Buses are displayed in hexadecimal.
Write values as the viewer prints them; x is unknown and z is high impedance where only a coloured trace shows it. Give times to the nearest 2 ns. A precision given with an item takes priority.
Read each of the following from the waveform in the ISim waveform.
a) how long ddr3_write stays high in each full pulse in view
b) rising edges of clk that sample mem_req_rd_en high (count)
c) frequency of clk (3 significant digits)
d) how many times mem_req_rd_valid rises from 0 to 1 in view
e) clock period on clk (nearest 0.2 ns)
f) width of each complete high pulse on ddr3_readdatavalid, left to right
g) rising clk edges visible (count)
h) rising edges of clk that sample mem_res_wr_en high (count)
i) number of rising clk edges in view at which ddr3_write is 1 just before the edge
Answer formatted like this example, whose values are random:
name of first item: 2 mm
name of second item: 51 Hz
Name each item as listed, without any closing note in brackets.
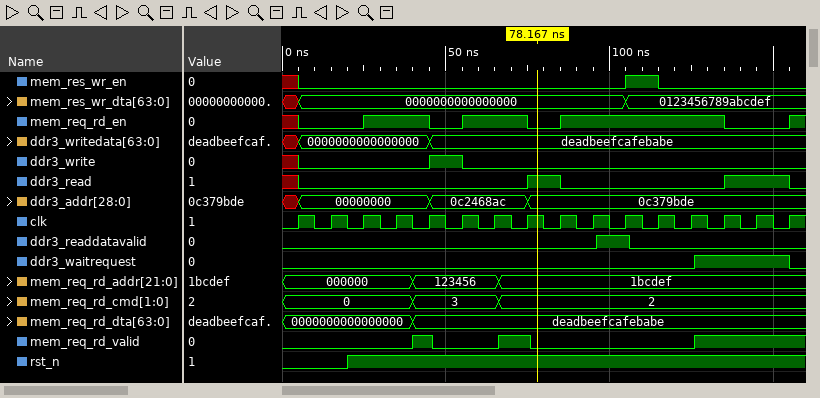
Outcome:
how long ddr3_write stays high in each full pulse in view: 10 ns
rising edges of clk that sample mem_req_rd_en high: 9
frequency of clk: 100 MHz
how many times mem_req_rd_valid rises from 0 to 1 in view: 3
clock period on clk: 10 ns
width of each complete high pulse on ddr3_readdatavalid, left to right: 10 ns
rising clk edges visible: 16
rising edges of clk that sample mem_res_wr_en high: 1
number of rising clk edges in view at which ddr3_write is 1 just before the edge: 1
